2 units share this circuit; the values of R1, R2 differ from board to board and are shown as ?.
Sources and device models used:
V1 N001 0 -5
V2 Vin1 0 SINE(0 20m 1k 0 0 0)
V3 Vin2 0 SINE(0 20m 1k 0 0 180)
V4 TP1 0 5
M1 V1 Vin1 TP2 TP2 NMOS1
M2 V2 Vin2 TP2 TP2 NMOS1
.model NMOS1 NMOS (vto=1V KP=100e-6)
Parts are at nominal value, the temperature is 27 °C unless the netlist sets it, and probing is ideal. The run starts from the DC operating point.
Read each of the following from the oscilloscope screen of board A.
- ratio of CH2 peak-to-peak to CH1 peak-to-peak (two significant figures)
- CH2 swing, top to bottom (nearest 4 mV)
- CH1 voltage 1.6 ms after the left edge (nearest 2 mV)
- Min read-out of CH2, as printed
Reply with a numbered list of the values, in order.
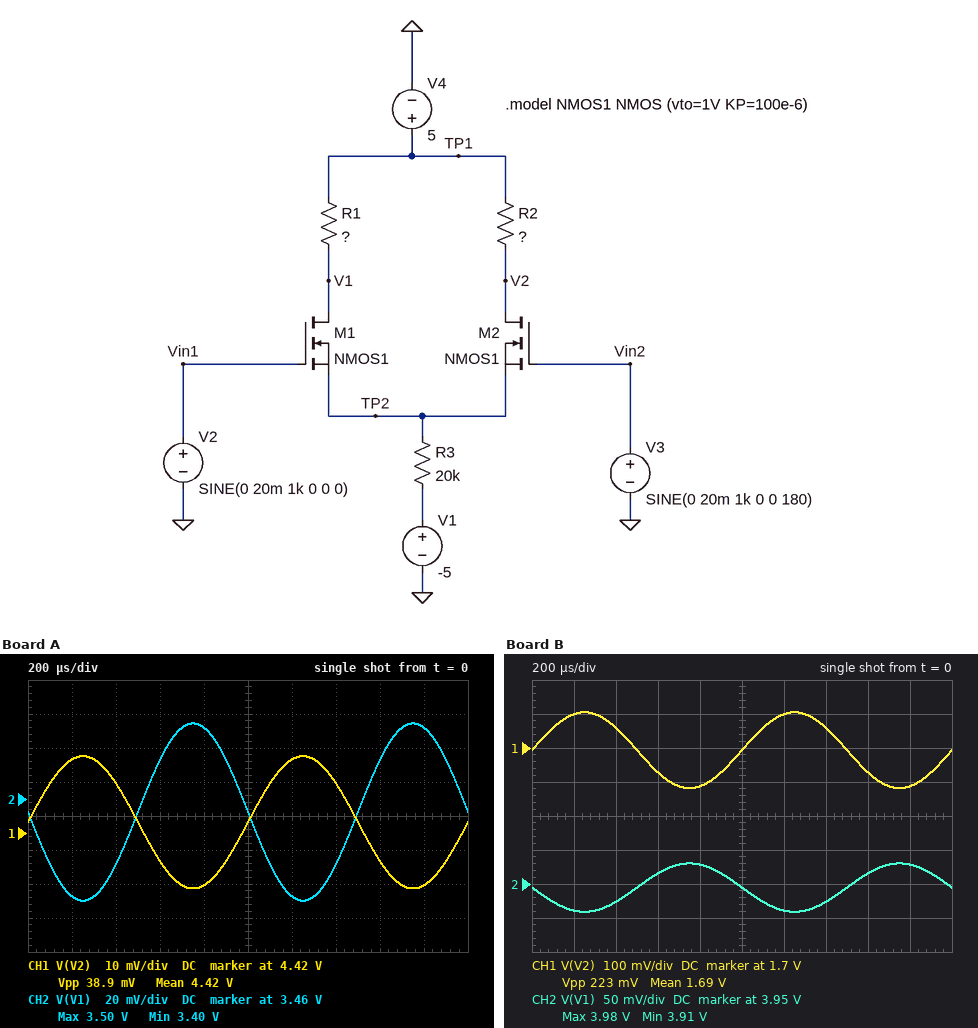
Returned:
1. 2.7
2. 104 mV
3. 4.412 V
4. 3.40 V
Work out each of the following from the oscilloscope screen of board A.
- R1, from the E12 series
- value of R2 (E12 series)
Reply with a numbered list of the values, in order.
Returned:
1. 22 kΩ
2. 8.2 kΩ
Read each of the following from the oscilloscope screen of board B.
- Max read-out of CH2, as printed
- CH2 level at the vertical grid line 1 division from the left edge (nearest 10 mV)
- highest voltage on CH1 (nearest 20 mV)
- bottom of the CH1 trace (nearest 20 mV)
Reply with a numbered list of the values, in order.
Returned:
1. 3.98 V
2. 3.91 V
3. 1.80 V
4. 1.58 V
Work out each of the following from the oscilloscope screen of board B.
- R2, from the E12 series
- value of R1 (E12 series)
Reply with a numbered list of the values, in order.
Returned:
1. 47 kΩ
2. 15 kΩ
